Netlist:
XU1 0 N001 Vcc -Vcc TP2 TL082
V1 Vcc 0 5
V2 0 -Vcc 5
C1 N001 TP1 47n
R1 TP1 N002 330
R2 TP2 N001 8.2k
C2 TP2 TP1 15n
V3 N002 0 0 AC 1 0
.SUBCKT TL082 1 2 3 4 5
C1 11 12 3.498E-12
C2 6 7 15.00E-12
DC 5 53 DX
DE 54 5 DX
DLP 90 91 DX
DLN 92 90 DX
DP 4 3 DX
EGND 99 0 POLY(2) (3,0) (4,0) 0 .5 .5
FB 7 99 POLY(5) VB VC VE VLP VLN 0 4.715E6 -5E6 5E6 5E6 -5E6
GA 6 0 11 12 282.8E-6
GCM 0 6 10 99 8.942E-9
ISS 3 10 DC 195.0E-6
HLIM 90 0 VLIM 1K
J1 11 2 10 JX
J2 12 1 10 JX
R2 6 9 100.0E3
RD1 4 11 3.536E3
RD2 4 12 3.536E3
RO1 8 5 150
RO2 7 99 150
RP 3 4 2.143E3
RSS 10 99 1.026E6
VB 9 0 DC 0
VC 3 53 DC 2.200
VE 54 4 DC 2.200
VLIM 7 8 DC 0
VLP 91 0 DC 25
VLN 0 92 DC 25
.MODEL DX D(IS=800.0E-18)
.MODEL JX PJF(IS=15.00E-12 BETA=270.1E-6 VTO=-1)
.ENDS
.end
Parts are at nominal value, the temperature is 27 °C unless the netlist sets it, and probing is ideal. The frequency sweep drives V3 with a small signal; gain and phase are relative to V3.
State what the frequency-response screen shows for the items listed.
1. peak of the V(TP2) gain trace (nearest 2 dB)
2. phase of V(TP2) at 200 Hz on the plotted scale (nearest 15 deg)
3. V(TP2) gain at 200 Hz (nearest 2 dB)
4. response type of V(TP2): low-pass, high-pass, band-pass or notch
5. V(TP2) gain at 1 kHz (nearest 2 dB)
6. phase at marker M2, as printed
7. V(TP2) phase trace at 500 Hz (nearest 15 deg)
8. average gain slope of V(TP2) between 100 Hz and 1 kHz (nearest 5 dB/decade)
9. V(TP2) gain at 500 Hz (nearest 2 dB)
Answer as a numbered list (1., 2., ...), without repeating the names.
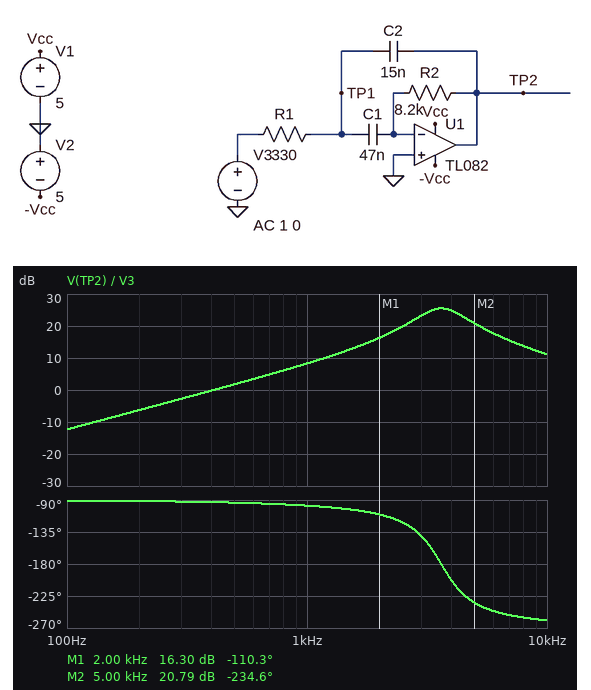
1. 26 dB
2. -90 deg
3. -6 dB
4. band-pass
5. 8 dB
6. -234.6 deg
7. -90 deg
8. 20 dB/decade
9. 2 dB
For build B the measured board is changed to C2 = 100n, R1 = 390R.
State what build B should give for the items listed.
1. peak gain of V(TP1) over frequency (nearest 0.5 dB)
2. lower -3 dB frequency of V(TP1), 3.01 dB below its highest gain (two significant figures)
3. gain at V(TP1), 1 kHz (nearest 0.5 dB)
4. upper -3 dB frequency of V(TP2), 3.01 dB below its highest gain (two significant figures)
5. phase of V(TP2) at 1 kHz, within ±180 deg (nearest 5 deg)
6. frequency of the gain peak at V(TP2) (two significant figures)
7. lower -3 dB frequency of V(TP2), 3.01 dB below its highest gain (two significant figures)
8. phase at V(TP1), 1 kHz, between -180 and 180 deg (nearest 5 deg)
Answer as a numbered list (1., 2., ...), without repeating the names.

1. 7.0 dB
2. 860 Hz
3. 5.5 dB
4. 1.6 kHz
5. -130 deg
6. 1.3 kHz
7. 1.0 kHz
8. -40 deg
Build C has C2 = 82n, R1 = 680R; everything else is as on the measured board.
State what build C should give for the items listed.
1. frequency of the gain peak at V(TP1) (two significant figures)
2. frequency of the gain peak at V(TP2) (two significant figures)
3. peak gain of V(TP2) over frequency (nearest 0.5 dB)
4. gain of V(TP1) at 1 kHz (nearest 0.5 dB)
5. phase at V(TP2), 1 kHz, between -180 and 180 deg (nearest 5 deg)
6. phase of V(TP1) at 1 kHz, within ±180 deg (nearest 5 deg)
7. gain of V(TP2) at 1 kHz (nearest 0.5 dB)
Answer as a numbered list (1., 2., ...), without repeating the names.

1. 980 Hz
2. 1.1 kHz
3. 13.0 dB
4. 5.0 dB
5. -165 deg
6. -75 deg
7. 12.5 dB
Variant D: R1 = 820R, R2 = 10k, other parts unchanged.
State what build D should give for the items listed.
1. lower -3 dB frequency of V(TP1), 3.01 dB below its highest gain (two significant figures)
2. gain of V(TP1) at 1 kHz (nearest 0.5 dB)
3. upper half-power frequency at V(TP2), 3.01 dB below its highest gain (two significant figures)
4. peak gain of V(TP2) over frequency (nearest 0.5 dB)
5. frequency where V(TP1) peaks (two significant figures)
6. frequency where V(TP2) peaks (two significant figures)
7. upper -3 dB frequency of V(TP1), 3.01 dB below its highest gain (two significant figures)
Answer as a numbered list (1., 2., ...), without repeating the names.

1. 800 Hz
2. 1.5 dB
3. 2.9 kHz
4. 19.5 dB
5. 1.8 kHz
6. 2.1 kHz
7. 2.5 kHz
